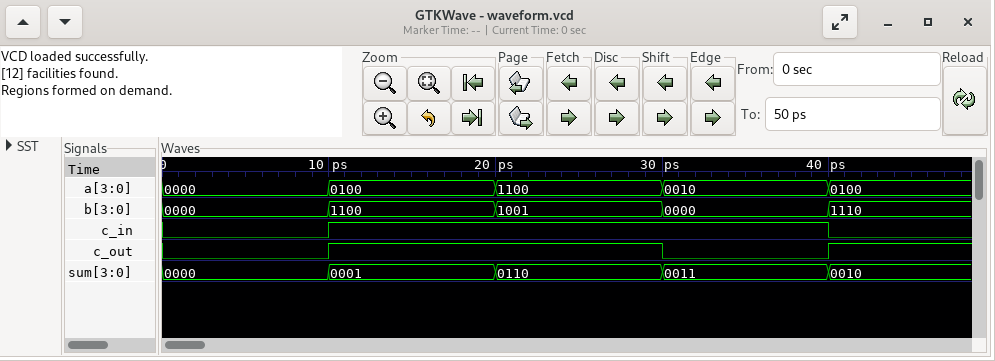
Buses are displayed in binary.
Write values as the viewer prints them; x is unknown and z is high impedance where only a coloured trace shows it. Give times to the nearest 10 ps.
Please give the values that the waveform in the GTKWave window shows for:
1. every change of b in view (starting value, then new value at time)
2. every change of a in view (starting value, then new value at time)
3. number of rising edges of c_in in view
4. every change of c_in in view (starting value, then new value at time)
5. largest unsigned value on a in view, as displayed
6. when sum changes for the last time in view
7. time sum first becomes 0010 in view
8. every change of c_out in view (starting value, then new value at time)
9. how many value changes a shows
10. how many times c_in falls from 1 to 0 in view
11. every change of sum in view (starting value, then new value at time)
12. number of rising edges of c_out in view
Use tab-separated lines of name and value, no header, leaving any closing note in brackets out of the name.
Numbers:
every change of b in view	0000, 1100 at 10 ps, 1001 at 20 ps, 0000 at 30 ps, 1110 at 40 ps
every change of a in view	0000, 0100 at 10 ps, 1100 at 20 ps, 0010 at 30 ps, 0100 at 40 ps
number of rising edges of c_in in view	1
every change of c_in in view	0, 1 at 10 ps, 0 at 40 ps
largest unsigned value on a in view, as displayed	1100
when sum changes for the last time in view	40 ps
time sum first becomes 0010 in view	40 ps
every change of c_out in view	0, 1 at 10 ps, 0 at 30 ps, 1 at 40 ps
how many value changes a shows	4
how many times c_in falls from 1 to 0 in view	1
every change of sum in view	0000, 0001 at 10 ps, 0110 at 20 ps, 0011 at 30 ps, 0010 at 40 ps
number of rising edges of c_out in view	2
